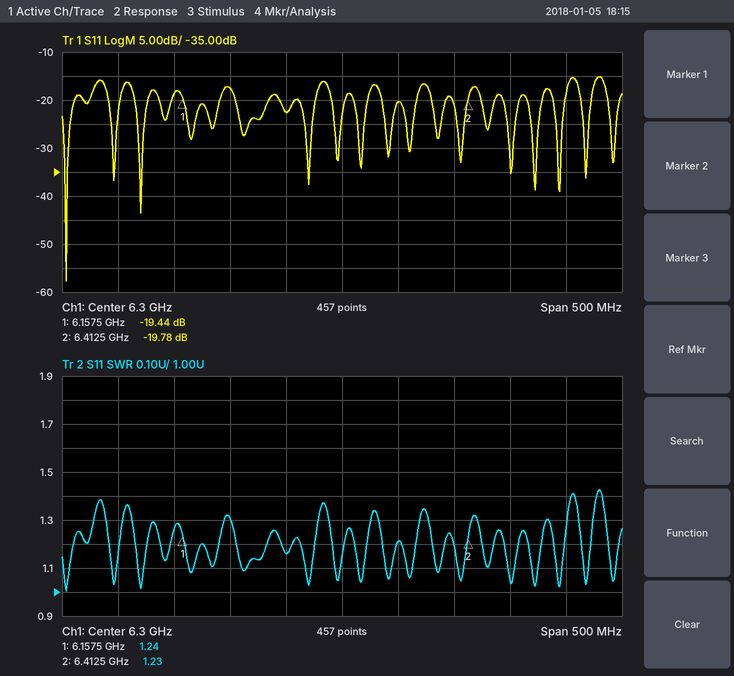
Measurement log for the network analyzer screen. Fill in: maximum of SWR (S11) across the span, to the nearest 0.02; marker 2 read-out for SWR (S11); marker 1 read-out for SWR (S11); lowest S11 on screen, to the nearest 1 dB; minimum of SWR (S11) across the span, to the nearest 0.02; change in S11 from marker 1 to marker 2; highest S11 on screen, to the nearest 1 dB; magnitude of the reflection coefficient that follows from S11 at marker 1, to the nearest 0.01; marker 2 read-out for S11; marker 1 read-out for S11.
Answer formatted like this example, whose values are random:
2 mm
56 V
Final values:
1.42
1.23
1.24
-58 dB
1.00
-0.34 dB
-15 dB
0.11
-19.78 dB
-19.44 dB
